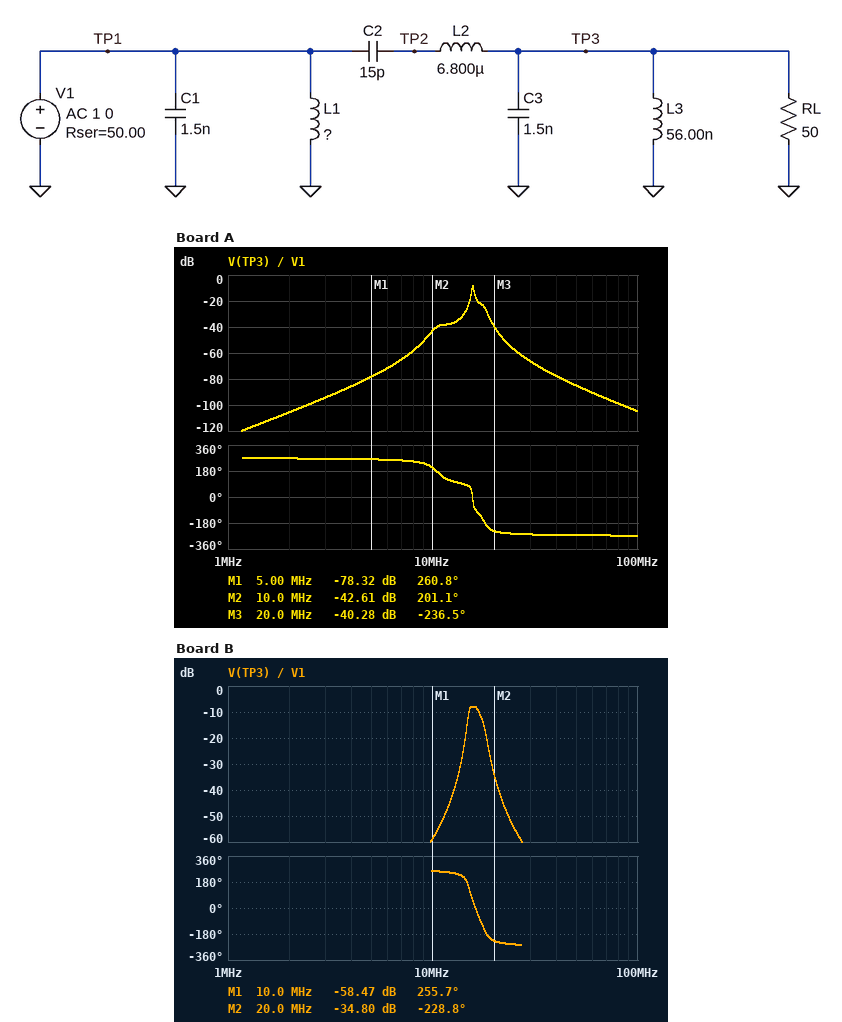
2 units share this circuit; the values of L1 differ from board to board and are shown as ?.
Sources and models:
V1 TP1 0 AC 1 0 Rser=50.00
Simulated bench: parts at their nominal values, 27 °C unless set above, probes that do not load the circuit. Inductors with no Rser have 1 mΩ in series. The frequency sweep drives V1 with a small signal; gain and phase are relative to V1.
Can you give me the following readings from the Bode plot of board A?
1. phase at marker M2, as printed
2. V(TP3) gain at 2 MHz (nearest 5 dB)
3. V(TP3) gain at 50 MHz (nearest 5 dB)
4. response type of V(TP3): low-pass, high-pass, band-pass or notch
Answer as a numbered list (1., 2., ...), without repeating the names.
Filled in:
1. 201.1 deg
2. -105 dB
3. -85 dB
4. band-pass
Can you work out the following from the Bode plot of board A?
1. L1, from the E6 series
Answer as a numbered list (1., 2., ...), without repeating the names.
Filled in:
1. 150 nH
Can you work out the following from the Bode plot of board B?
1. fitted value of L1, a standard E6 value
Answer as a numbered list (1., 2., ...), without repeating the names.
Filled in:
1. 68 nH
